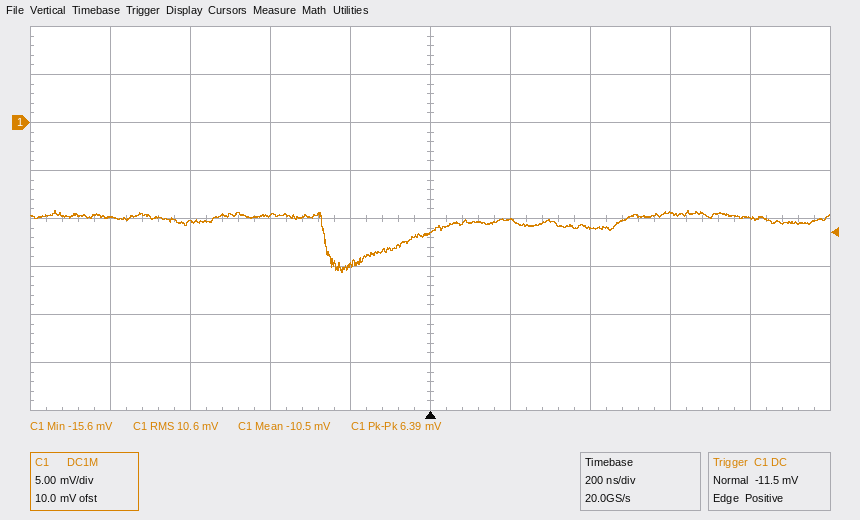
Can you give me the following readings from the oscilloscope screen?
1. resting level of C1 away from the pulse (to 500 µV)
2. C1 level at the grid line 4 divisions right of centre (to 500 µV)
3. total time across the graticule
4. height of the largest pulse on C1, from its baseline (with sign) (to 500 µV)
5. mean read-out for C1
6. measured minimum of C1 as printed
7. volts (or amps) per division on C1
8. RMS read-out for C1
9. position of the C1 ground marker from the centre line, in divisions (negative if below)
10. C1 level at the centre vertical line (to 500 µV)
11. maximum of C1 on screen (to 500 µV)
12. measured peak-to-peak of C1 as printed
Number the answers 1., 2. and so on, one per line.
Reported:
1. -10.0 mV
2. -10.0 mV
3. 2 µs
4. -5.5 mV
5. -10.5 mV
6. -15.6 mV
7. 5 mV
8. 10.6 mV
9. +2.0 div
10. -11.5 mV
11. -9.0 mV
12. 6.39 mV
